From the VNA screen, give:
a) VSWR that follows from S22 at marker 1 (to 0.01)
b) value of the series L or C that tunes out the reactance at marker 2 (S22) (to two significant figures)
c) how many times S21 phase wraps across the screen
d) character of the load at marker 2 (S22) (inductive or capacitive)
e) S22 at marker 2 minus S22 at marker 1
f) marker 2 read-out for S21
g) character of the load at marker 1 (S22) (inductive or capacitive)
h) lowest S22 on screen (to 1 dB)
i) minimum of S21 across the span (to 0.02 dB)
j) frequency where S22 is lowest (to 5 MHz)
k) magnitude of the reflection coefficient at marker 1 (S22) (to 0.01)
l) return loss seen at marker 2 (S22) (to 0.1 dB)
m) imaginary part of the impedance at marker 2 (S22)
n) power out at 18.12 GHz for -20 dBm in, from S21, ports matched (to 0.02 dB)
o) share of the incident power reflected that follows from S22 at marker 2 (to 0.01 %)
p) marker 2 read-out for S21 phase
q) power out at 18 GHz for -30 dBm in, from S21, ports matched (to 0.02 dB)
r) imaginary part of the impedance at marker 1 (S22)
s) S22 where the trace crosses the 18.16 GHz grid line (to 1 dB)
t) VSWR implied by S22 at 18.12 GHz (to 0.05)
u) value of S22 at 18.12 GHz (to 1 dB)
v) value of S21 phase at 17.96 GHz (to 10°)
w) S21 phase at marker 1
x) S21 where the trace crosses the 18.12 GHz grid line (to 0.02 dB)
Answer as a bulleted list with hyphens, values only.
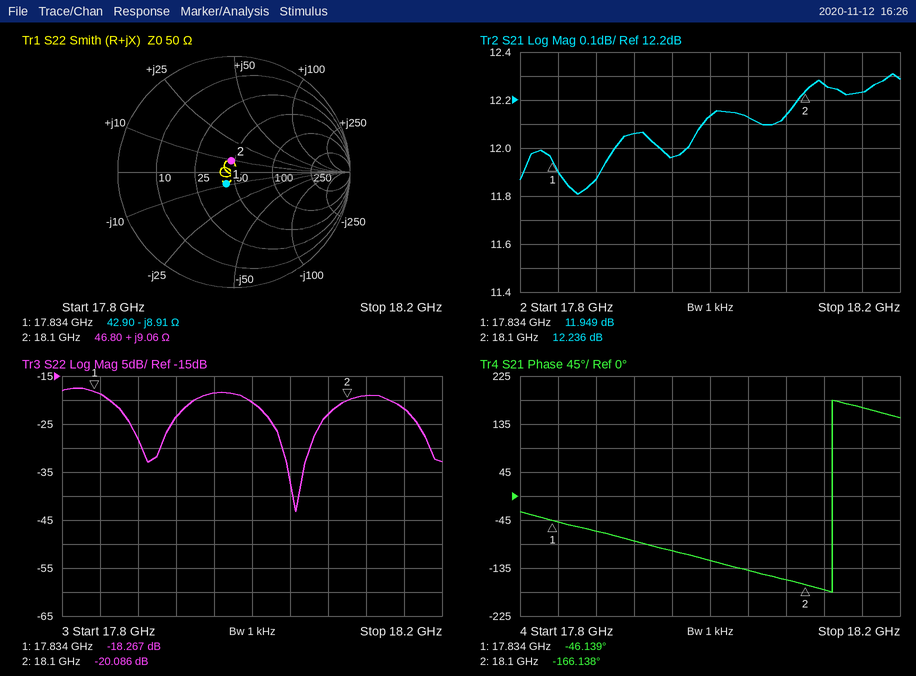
- 1.28
- 970 fF
- 1
- inductive
- -1.819 dB
- 12.236 dB
- capacitive
- -43 dB
- 11.80 dB
- 18.045 GHz
- 0.12
- 20.1 dB
- +9.06 Ω
- -7.74 dBm
- 0.98 %
- -166.138°
- -17.86 dBm
- -8.91 Ω
- -22 dB
- 1.25
- -19 dB
- -100°
- -46.139°
- 12.26 dB
